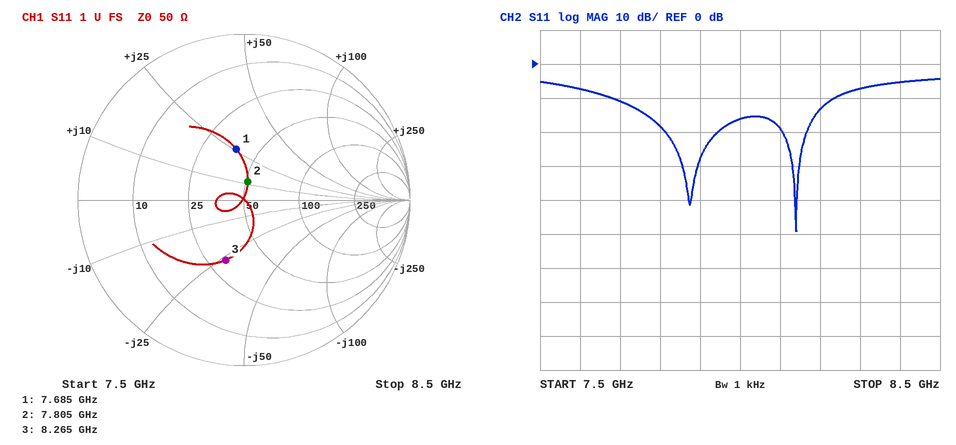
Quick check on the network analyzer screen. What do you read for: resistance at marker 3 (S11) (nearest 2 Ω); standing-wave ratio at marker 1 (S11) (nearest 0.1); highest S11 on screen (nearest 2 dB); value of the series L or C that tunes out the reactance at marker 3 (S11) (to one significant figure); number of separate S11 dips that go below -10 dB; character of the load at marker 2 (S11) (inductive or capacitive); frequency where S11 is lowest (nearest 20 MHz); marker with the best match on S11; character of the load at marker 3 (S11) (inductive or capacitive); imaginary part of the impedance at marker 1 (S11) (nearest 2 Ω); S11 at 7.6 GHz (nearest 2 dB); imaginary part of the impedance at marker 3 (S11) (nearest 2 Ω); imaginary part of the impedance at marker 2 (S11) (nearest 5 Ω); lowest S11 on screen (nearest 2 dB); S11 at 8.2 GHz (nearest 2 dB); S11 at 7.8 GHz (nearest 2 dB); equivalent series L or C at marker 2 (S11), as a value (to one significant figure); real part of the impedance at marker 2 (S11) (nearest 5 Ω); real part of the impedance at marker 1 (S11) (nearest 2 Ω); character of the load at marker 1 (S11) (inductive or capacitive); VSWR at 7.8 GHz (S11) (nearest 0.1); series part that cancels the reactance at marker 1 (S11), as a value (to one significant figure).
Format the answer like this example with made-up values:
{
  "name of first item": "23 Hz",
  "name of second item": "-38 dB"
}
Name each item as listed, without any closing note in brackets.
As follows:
{
  "resistance at marker 3 (S11)": "32 Ω",
  "standing-wave ratio at marker 1 (S11)": "1.9",
  "highest S11 on screen": "-4 dB",
  "value of the series L or C that tunes out the reactance at marker 3 (S11)": "500 pH",
  "number of separate S11 dips that go below -10 dB": "2",
  "character of the load at marker 2 (S11)": "inductive",
  "frequency where S11 is lowest": "8.14 GHz",
  "marker with the best match on S11": "marker 2",
  "character of the load at marker 3 (S11)": "capacitive",
  "imaginary part of the impedance at marker 1 (S11)": "+26 Ω",
  "S11 at 7.6 GHz": "-8 dB",
  "imaginary part of the impedance at marker 3 (S11)": "-26 Ω",
  "imaginary part of the impedance at marker 2 (S11)": "+10 Ω",
  "lowest S11 on screen": "-50 dB",
  "S11 at 8.2 GHz": "-14 dB",
  "S11 at 7.8 GHz": "-18 dB",
  "equivalent series L or C at marker 2 (S11), as a value": "200 pH",
  "real part of the impedance at marker 2 (S11)": "50 Ω",
  "real part of the impedance at marker 1 (S11)": "38 Ω",
  "character of the load at marker 1 (S11)": "inductive",
  "VSWR at 7.8 GHz (S11)": "1.3",
  "series part that cancels the reactance at marker 1 (S11), as a value": "800 fF"
}
